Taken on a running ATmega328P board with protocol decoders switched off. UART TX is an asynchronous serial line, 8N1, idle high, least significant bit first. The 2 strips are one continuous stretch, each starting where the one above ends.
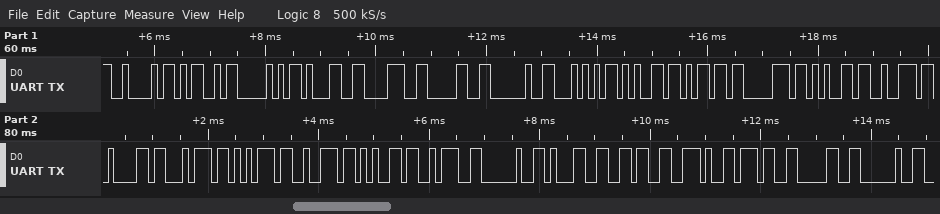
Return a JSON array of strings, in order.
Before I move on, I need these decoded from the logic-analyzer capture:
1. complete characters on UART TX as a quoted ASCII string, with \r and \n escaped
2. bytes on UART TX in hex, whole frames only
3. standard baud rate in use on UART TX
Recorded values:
["\"BMP180 Temperature: 16.70 \"", "42 4D 50 31 38 30 20 54 65 6D 70 65 72 61 74 75 72 65 3A 20 31 36 2E 37 30 20", "9600 baud"]
